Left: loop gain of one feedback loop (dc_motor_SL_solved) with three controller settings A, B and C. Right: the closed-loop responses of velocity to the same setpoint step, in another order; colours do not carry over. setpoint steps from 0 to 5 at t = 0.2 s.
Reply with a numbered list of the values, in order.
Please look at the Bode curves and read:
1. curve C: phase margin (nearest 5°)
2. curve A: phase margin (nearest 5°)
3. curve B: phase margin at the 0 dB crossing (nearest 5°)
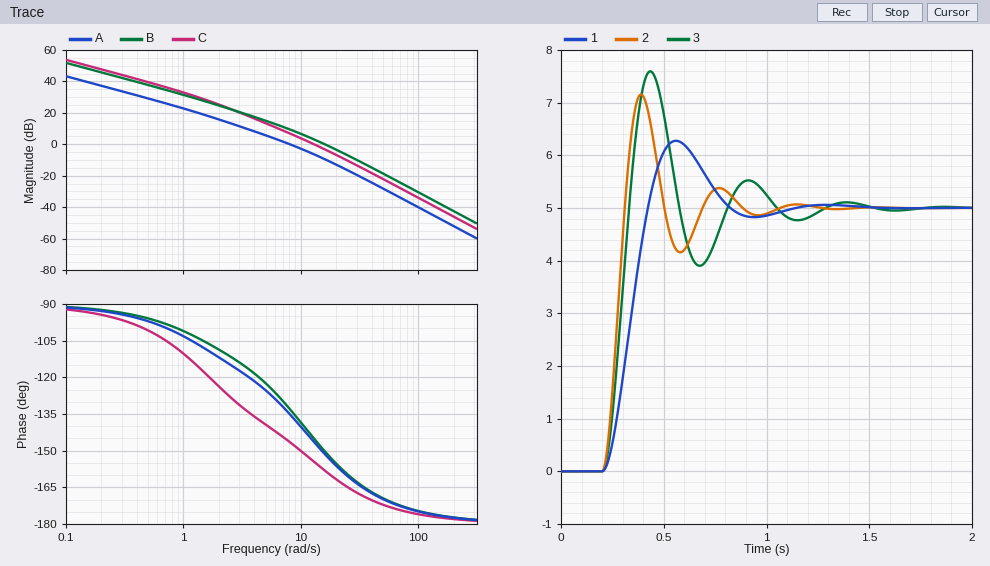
1. 25°
2. 45°
3. 30°
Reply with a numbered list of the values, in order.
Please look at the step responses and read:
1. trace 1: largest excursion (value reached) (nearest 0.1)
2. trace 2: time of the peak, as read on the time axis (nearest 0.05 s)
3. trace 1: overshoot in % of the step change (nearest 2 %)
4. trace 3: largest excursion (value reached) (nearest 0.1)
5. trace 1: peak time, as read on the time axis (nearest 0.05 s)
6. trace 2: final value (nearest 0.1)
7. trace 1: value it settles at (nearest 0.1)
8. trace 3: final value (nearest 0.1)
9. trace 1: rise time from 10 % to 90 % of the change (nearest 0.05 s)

1. 6.3
2. 0.40 s
3. 26 %
4. 7.6
5. 0.55 s
6. 5.0
7. 5.0
8. 5.0
9. 0.15 s
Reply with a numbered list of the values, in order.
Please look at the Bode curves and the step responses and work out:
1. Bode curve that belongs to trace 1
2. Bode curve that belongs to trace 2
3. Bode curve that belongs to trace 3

1. A
2. B
3. C
